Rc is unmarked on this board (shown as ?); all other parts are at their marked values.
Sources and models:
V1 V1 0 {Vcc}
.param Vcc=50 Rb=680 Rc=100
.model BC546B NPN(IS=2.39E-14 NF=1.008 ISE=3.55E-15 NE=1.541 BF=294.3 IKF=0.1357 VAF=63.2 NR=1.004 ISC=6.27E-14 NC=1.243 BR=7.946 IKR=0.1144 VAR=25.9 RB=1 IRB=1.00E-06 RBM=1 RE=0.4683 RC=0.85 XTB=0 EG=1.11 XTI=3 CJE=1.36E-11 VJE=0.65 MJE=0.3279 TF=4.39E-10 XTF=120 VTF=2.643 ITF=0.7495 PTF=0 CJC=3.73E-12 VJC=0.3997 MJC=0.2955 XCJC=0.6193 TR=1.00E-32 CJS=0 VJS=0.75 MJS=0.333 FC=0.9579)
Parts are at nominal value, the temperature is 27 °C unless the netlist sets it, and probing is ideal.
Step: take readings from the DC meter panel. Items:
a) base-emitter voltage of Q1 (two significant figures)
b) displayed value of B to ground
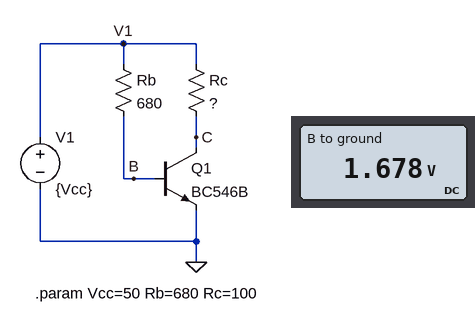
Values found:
1.7 V
1.678 V
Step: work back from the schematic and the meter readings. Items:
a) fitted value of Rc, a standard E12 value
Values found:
33 Ω
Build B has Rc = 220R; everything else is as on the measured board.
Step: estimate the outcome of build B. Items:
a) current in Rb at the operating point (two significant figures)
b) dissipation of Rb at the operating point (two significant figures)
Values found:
72 mA
3.5 W
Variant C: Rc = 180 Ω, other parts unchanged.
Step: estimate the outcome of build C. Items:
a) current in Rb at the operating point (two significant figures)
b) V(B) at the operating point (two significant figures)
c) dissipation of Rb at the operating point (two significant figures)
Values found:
72 mA
1.1 V
3.5 W
